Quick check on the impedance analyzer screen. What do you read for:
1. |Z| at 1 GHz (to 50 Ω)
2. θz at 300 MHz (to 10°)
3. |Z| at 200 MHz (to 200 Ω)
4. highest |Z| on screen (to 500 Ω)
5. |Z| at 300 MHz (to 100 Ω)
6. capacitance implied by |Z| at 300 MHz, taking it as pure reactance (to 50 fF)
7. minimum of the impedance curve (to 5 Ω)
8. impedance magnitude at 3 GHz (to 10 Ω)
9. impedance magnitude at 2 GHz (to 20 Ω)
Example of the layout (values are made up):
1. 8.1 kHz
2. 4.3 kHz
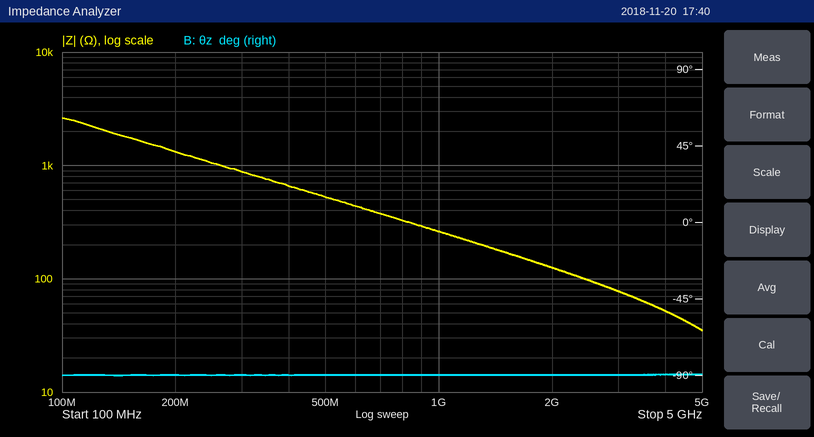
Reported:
1. 250 Ω
2. -90°
3. 1.4 kΩ
4. 2.5 kΩ
5. 900 Ω
6. 600 fF
7. 35 Ω
8. 80 Ω
9. 120 Ω
